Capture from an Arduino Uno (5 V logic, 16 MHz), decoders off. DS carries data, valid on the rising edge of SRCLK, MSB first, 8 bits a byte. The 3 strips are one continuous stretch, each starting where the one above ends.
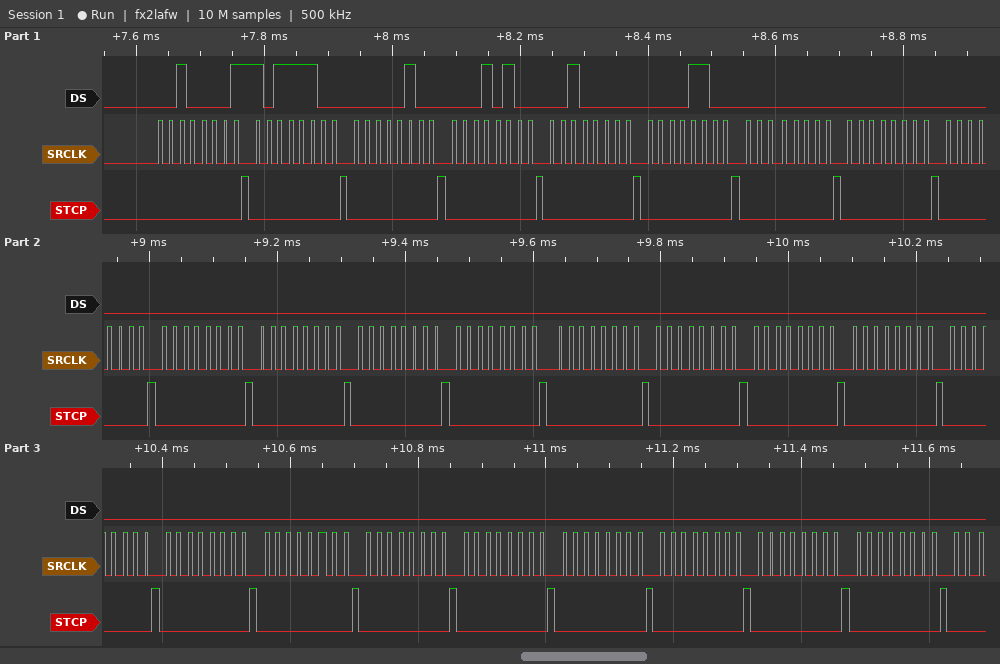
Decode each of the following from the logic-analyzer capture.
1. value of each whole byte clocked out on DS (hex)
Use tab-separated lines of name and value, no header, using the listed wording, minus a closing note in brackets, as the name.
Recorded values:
value of each whole byte clocked out on DS	0x21 0xBC 0x04 0x14 0x20 0x0C 0x00 0x00 0x00 0x00 0x00 0x00 0x00 0x00 0x00 0x00 0x00 0x00 0x00 0x00 0x00 0x00 0x00 0x00 0x00 0x00
